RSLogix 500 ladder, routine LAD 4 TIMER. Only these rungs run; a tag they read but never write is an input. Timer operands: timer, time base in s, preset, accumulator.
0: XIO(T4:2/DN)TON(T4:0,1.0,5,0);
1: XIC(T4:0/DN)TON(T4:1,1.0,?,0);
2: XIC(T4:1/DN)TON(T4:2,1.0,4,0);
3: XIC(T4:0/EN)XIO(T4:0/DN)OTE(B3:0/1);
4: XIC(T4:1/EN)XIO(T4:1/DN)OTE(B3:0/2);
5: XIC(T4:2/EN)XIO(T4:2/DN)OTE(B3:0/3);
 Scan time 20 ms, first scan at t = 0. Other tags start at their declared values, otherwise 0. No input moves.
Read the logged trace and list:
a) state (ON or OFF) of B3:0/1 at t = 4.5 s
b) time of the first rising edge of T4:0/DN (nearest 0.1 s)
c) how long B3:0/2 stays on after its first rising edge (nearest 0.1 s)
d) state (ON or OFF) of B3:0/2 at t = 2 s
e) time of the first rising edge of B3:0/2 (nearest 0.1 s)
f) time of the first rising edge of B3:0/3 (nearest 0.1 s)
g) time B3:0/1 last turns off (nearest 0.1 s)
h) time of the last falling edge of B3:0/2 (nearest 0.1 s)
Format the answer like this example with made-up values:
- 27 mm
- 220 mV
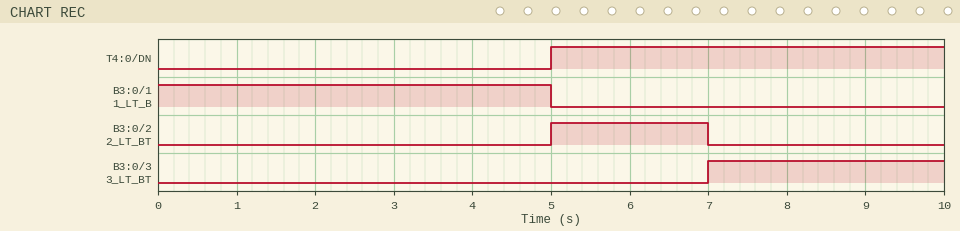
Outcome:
- ON
- 5.0 s
- 2.0 s
- OFF
- 5.0 s
- 7.0 s
- 5.0 s
- 7.0 s
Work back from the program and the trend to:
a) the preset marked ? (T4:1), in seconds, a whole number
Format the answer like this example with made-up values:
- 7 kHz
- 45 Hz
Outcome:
- 2 s
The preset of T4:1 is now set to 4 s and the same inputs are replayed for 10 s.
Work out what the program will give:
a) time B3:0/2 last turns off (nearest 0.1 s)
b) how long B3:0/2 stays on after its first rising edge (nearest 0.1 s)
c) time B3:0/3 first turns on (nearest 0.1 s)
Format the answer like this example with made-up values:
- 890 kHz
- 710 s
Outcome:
- 9.0 s
- 4.0 s
- 9.0 s
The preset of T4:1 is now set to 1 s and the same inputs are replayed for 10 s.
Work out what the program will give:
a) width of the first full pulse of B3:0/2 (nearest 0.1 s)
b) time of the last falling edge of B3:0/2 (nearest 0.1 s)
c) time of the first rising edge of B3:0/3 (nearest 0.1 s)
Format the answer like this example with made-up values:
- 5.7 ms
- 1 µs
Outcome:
- 1.0 s
- 6.0 s
- 6.0 s
